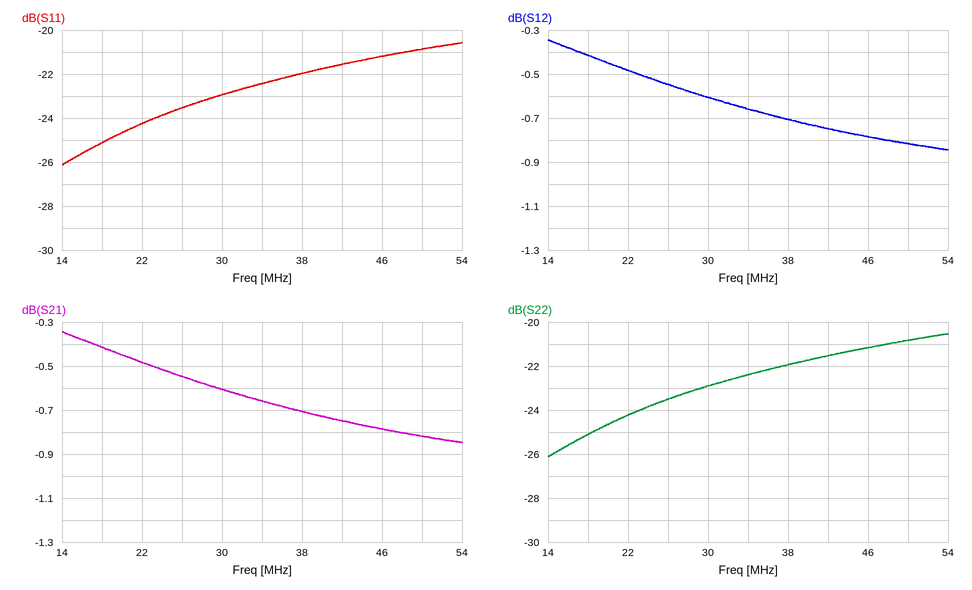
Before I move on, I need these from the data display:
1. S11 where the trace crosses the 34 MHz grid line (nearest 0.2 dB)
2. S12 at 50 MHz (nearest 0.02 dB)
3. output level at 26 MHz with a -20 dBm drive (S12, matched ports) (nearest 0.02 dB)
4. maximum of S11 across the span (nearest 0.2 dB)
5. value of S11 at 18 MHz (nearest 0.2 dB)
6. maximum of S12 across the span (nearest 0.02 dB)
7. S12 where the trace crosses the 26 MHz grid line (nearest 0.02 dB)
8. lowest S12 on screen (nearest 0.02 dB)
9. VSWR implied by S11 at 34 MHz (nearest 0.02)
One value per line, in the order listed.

-22.4 dB
-0.82 dB
-20.54 dBm
-20.6 dB
-25.2 dB
-0.34 dB
-0.54 dB
-0.84 dB
1.16
